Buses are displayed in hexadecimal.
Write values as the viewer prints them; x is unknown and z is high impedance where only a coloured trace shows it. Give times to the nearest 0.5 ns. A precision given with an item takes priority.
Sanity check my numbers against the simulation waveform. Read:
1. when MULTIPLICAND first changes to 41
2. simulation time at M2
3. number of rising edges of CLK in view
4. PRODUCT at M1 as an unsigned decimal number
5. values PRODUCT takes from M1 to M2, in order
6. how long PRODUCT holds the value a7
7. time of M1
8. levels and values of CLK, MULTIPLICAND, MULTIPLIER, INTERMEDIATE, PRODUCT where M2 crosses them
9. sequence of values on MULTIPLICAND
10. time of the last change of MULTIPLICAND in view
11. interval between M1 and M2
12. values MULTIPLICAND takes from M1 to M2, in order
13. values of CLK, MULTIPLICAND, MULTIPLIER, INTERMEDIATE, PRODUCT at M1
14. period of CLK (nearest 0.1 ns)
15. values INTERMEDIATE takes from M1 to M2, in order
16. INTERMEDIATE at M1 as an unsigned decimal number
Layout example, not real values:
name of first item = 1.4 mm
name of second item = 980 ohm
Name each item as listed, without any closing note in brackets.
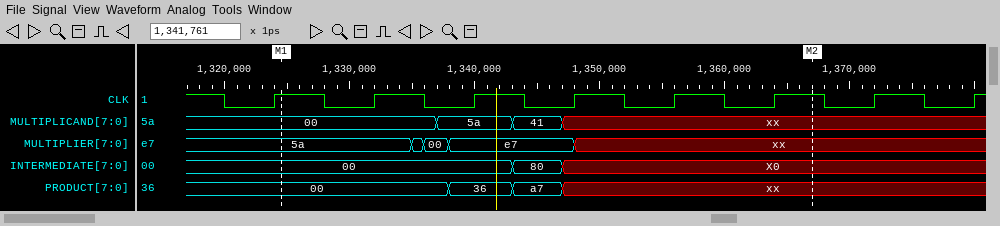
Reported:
when MULTIPLICAND first changes to 41 = 1343 ns
simulation time at M2 = 1367 ns
number of rising edges of CLK in view = 8
PRODUCT at M1 as an unsigned decimal number = 0
values PRODUCT takes from M1 to M2, in order = 00, 36, a7, xx
how long PRODUCT holds the value a7 = 4 ns
time of M1 = 1324.5 ns
levels and values of CLK, MULTIPLICAND, MULTIPLIER, INTERMEDIATE, PRODUCT where M2 crosses them = CLK=1, MULTIPLICAND=xx, MULTIPLIER=xx, INTERMEDIATE=X0, PRODUCT=xx
sequence of values on MULTIPLICAND = 00, 5a, 41, xx
time of the last change of MULTIPLICAND in view = 1347 ns
interval between M1 and M2 = 42.5 ns
values MULTIPLICAND takes from M1 to M2, in order = 00, 5a, 41, xx
values of CLK, MULTIPLICAND, MULTIPLIER, INTERMEDIATE, PRODUCT at M1 = CLK=1, MULTIPLICAND=00, MULTIPLIER=5a, INTERMEDIATE=00, PRODUCT=00
period of CLK = 8 ns
values INTERMEDIATE takes from M1 to M2, in order = 00, 80, X0
INTERMEDIATE at M1 as an unsigned decimal number = 0
